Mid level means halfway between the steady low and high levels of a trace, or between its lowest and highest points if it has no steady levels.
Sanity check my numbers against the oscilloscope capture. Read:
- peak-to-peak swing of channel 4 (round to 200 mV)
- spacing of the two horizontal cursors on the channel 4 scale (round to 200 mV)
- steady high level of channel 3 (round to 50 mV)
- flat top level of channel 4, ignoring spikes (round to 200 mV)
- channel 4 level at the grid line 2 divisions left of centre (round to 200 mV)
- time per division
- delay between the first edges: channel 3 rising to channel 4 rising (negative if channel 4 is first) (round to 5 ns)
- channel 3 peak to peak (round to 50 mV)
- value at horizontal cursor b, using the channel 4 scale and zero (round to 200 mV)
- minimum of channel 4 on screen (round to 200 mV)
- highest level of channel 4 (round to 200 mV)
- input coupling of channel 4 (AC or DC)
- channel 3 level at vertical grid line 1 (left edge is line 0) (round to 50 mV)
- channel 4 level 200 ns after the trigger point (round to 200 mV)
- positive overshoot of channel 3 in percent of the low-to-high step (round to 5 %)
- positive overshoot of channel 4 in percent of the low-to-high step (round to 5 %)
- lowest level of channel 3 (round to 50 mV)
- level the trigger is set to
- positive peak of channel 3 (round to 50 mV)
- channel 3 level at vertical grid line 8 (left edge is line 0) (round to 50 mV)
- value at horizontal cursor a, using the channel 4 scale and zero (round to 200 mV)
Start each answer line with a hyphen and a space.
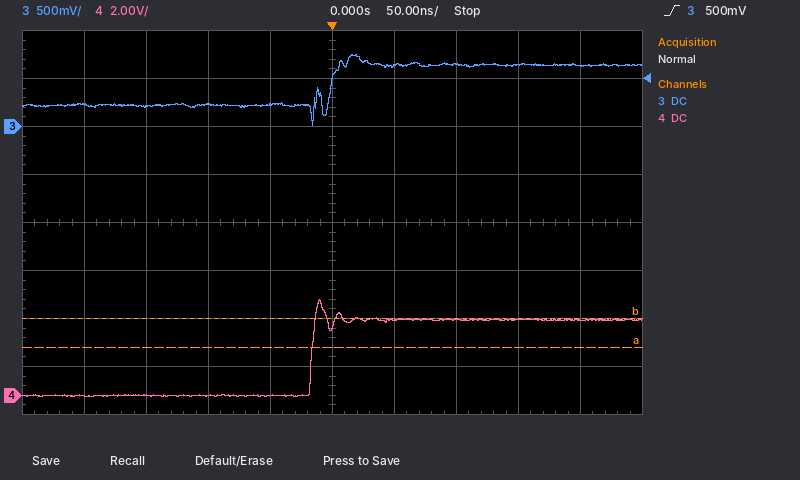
- 4.0 V
- 1.2 V
- 650 mV
- 3.2 V
- 0.0 V
- 50 ns
- -15 ns
- 750 mV
- 3.2 V
- 0.0 V
- 4.0 V
- DC
- 250 mV
- 3.2 V
- 25 %
- 25 %
- 0 mV
- 500 mV
- 750 mV
- 650 mV
- 2.0 V
